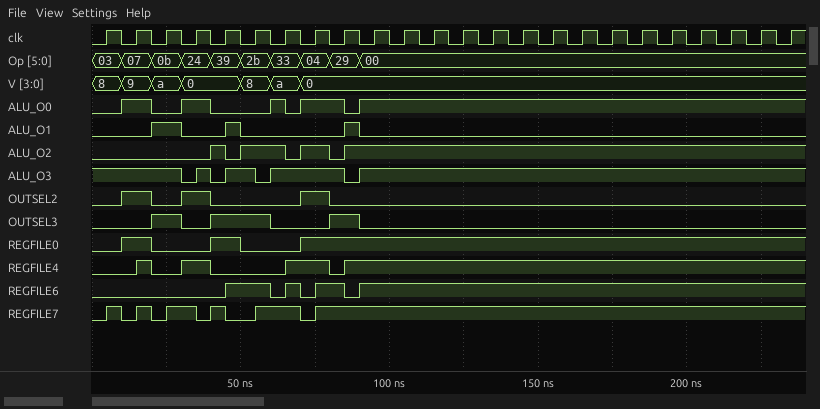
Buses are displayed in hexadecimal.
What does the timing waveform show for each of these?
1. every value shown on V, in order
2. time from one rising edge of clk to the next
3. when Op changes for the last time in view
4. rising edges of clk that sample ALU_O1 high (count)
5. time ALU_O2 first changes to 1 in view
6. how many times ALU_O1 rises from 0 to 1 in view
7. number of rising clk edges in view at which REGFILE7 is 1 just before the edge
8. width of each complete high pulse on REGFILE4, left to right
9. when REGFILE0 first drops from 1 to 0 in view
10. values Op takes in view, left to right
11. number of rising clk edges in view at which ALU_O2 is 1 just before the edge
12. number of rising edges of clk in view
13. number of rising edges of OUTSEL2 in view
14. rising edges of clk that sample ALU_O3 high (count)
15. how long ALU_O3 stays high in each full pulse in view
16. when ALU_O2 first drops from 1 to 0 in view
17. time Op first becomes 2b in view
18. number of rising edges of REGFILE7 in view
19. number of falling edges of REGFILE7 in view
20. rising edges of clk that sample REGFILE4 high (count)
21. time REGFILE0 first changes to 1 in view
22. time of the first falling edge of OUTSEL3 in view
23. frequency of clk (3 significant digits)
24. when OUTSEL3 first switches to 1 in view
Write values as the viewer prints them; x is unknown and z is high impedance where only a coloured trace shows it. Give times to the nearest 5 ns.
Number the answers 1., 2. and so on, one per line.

1. 8, 9, a, 0, 8, a, 0
2. 10 ns
3. 90 ns
4. 1
5. 40 ns
6. 3
7. 19
8. 5 ns, 10 ns, 15 ns
9. 20 ns
10. 03, 07, 0b, 24, 39, 2b, 33, 04, 29, 00
11. 19
12. 24
13. 3
14. 22
15. 5 ns, 10 ns, 25 ns
16. 45 ns
17. 50 ns
18. 6
19. 5
20. 17
21. 10 ns
22. 30 ns
23. 100 MHz
24. 20 ns
